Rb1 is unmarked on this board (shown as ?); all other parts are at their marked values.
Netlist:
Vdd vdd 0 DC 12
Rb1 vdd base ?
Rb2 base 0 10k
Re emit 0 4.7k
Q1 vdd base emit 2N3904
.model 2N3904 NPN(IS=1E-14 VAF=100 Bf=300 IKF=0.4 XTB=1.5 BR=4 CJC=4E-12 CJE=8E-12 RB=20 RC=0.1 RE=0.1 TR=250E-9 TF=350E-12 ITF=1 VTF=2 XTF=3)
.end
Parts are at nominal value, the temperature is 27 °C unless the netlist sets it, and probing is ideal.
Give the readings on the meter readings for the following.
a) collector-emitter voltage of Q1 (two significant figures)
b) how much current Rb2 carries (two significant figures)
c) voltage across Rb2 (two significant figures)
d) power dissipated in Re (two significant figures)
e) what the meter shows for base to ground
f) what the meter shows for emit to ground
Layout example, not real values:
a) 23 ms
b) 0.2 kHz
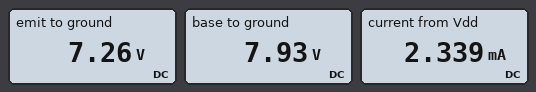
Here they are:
a) 4.7 V
b) 790 µA
c) 7.9 V
d) 11 mW
e) 7.93 V
f) 7.26 V
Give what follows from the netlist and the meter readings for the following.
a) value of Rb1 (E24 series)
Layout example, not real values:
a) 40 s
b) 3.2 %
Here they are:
a) 5.1 kΩ
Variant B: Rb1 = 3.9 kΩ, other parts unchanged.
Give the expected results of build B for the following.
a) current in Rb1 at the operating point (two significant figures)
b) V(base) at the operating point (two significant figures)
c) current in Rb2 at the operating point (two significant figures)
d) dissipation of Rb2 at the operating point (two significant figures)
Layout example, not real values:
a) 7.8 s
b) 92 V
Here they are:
a) 870 µA
b) 8.6 V
c) 860 µA
d) 7.4 mW
